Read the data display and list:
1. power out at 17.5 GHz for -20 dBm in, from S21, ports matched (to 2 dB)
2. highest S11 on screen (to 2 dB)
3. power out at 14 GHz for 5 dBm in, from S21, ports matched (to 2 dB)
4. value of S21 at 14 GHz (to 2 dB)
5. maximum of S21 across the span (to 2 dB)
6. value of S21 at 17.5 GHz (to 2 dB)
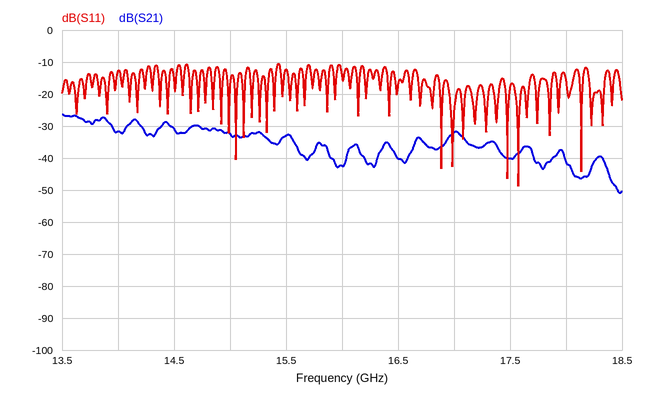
-60 dBm
-10 dB
-26 dBm
-32 dB
-26 dB
-40 dB
